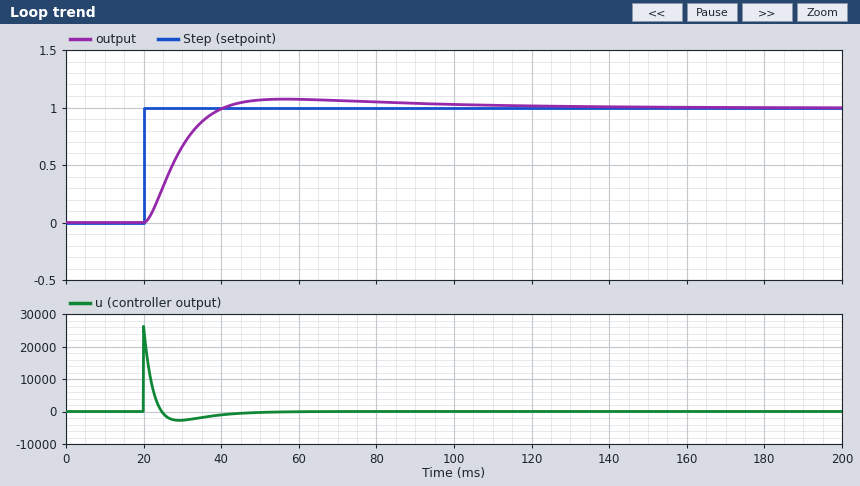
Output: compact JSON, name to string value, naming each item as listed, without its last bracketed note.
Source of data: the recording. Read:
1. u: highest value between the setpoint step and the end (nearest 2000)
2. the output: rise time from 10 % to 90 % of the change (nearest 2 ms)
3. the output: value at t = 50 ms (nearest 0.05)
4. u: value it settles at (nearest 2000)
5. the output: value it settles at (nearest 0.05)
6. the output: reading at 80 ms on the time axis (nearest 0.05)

{"u: highest value between the setpoint step and the end": "26000", "the output: rise time from 10 % to 90 % of the change": "14 ms", "the output: value at t = 50 ms": "1.05", "u: value it settles at": "0", "the output: value it settles at": "1.00", "the output: reading at 80 ms on the time axis": "1.05"}
